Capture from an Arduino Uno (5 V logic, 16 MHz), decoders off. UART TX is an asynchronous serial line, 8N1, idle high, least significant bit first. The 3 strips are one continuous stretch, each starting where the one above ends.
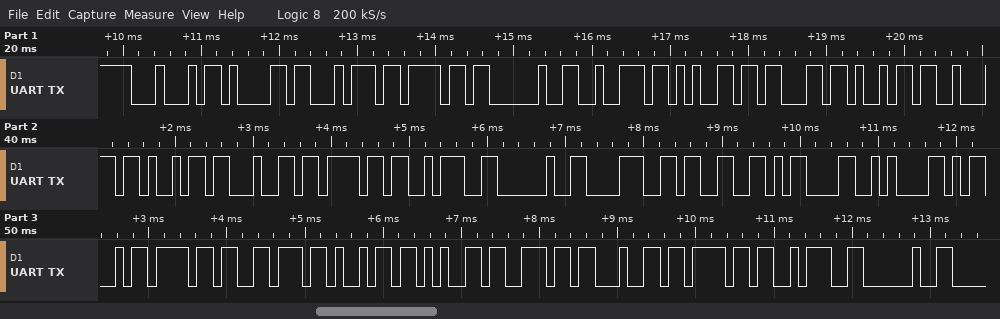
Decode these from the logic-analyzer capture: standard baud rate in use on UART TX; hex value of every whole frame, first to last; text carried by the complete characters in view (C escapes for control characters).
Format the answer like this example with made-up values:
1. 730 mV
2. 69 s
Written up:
1. 9600 baud
2. 44 61 74 6F 20 72 65 63 69 62 69 64 6F 3A 20 38 33 0D 0A 4D 6F 76 69 65 6E 64 6F 3A 20
3. "Dato recibido: 83\r\nMoviendo: "
